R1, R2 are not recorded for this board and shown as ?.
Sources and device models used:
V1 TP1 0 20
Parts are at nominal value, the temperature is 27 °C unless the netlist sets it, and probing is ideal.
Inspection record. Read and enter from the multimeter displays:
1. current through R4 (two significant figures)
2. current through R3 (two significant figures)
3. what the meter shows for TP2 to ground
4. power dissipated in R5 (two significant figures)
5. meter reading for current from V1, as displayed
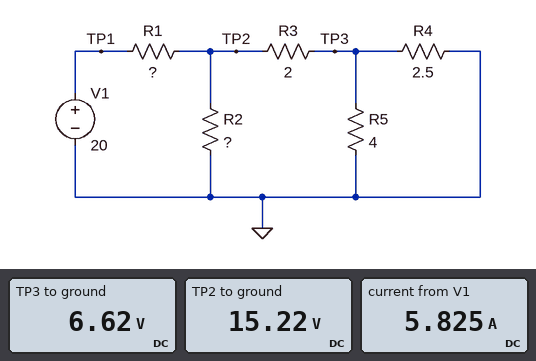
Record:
2.6 A
4.3 A
15.22 V
11 W
5.825 A
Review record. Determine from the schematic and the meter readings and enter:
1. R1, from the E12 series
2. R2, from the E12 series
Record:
0.82 Ω
10 Ω
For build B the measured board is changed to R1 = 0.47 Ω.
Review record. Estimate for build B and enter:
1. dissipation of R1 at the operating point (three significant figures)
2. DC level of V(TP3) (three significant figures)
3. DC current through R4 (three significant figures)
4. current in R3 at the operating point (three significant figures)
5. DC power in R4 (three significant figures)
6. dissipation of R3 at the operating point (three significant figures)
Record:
19.8 W
7.37 V
2.95 A
4.79 A
21.7 W
45.9 W
